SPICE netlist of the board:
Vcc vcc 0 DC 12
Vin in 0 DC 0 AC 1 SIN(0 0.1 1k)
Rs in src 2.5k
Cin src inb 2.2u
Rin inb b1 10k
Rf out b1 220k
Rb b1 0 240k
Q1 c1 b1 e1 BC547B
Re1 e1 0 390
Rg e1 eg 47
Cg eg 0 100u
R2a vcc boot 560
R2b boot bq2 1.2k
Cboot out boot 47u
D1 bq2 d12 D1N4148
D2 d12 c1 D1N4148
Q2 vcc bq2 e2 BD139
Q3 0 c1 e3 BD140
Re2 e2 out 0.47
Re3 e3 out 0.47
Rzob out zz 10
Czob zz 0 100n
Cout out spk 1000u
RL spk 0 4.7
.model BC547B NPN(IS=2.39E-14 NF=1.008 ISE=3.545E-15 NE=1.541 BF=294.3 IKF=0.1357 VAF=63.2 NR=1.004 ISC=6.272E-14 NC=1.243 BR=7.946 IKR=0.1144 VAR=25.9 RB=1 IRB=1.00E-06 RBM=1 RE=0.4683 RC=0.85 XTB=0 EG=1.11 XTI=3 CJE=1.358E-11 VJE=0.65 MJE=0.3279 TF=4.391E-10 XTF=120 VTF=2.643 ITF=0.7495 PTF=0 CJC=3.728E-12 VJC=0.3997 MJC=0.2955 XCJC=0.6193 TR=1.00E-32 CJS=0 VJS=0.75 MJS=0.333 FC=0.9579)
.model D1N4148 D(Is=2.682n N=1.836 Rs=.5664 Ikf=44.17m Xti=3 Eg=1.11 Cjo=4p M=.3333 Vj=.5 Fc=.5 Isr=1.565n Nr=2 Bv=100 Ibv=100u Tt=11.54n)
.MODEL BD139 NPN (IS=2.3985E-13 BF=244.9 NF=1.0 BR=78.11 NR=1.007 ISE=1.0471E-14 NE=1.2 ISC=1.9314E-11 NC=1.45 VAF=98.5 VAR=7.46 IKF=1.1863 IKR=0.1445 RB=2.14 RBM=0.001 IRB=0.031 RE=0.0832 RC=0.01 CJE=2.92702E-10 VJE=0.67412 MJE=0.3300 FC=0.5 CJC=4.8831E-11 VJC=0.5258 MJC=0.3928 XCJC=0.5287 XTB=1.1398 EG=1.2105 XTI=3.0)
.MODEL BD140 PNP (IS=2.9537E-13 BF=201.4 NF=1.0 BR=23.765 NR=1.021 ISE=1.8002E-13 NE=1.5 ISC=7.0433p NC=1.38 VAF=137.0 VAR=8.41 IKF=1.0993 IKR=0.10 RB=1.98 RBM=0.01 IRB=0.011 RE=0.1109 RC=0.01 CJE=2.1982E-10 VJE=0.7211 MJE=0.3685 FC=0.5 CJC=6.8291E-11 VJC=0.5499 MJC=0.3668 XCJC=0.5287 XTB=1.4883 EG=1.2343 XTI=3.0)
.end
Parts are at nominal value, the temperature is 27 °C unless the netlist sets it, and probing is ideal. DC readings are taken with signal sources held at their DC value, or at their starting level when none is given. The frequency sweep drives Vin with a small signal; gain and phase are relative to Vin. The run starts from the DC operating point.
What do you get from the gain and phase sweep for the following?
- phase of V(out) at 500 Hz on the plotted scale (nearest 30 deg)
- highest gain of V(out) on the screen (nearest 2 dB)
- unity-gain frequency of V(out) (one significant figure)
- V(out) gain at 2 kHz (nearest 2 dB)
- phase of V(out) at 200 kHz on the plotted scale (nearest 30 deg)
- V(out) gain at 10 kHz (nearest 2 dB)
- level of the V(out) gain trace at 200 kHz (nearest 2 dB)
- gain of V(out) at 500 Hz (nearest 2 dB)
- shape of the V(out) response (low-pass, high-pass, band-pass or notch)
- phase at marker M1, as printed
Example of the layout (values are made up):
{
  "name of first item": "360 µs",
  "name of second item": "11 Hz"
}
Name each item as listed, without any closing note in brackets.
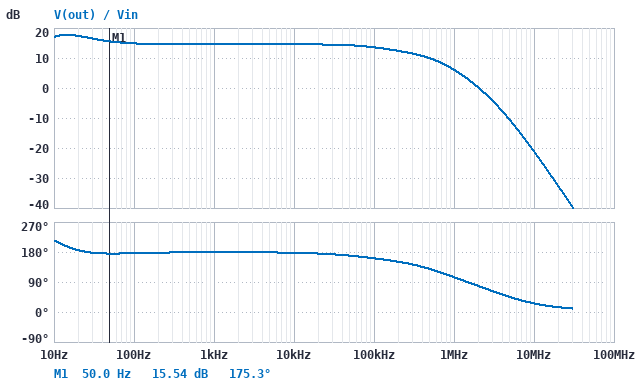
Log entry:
{
  "phase of V(out) at 500 Hz on the plotted scale": "180 deg",
  "highest gain of V(out) on the screen": "18 dB",
  "unity-gain frequency of V(out)": "2 MHz",
  "V(out) gain at 2 kHz": "14 dB",
  "phase of V(out) at 200 kHz on the plotted scale": "150 deg",
  "V(out) gain at 10 kHz": "14 dB",
  "level of the V(out) gain trace at 200 kHz": "12 dB",
  "gain of V(out) at 500 Hz": "14 dB",
  "shape of the V(out) response": "low-pass",
  "phase at marker M1, as printed": "175.3 deg"
}
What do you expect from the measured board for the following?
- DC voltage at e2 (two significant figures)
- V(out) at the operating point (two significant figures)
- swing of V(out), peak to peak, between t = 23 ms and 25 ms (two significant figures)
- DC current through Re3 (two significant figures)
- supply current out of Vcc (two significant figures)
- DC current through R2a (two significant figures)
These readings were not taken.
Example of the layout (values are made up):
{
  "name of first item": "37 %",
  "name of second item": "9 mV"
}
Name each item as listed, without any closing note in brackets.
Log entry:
{
  "DC voltage at e2": "5.9 V",
  "V(out) at the operating point": "5.9 V",
  "swing of V(out), peak to peak, between t = 23 ms and 25 ms": "1.0 V",
  "DC current through Re3": "25 mA",
  "supply current out of Vcc": "28 mA",
  "DC current through R2a": "3.1 mA"
}
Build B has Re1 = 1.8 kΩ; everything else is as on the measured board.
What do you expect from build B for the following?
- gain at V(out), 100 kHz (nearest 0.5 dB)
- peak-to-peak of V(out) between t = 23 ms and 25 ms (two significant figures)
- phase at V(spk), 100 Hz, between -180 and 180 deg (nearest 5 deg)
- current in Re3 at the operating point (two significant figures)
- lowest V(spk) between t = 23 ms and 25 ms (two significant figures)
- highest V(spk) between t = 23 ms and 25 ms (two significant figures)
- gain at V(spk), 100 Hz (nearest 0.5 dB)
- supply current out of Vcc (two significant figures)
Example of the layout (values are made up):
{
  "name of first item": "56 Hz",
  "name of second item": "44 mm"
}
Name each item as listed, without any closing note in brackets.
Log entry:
{
  "gain at V(out), 100 kHz": "12.5 dB",
  "peak-to-peak of V(out) between t = 23 ms and 25 ms": "940 mV",
  "phase at V(spk), 100 Hz, between -180 and 180 deg": "-165 deg",
  "current in Re3 at the operating point": "10 mA",
  "lowest V(spk) between t = 23 ms and 25 ms": "-470 mV",
  "highest V(spk) between t = 23 ms and 25 ms": "470 mV",
  "gain at V(spk), 100 Hz": "13.5 dB",
  "supply current out of Vcc": "12 mA"
}
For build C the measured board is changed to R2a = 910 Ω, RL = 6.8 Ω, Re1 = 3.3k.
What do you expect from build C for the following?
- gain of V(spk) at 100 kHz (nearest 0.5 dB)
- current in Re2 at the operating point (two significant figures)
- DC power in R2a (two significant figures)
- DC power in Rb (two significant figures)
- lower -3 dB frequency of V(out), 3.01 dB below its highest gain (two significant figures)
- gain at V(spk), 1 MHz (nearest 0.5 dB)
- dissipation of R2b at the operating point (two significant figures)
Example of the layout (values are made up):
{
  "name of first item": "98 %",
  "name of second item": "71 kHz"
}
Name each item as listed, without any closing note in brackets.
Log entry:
{
  "gain of V(spk) at 100 kHz": "13.0 dB",
  "current in Re2 at the operating point": "4.9 mA",
  "DC power in R2a": "1.1 mW",
  "DC power in Rb": "77 µW",
  "lower -3 dB frequency of V(out), 3.01 dB below its highest gain": "5.3 Hz",
  "gain at V(spk), 1 MHz": "0 dB",
  "dissipation of R2b at the operating point": "1.5 mW"
}
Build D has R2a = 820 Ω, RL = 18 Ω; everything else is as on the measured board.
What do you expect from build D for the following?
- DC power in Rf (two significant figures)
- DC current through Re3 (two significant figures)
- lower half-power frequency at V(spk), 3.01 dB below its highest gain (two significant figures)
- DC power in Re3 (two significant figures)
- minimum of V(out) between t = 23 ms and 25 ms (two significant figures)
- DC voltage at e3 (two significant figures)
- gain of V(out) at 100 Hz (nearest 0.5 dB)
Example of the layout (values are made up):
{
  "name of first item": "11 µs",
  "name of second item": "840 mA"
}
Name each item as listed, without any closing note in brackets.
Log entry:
{
  "DC power in Rf": "65 µW",
  "DC current through Re3": "22 mA",
  "lower half-power frequency at V(spk), 3.01 dB below its highest gain": "15 Hz",
  "DC power in Re3": "230 µW",
  "minimum of V(out) between t = 23 ms and 25 ms": "4.5 V",
  "DC voltage at e3": "5.6 V",
  "gain of V(out) at 100 Hz": "20.5 dB"
}
